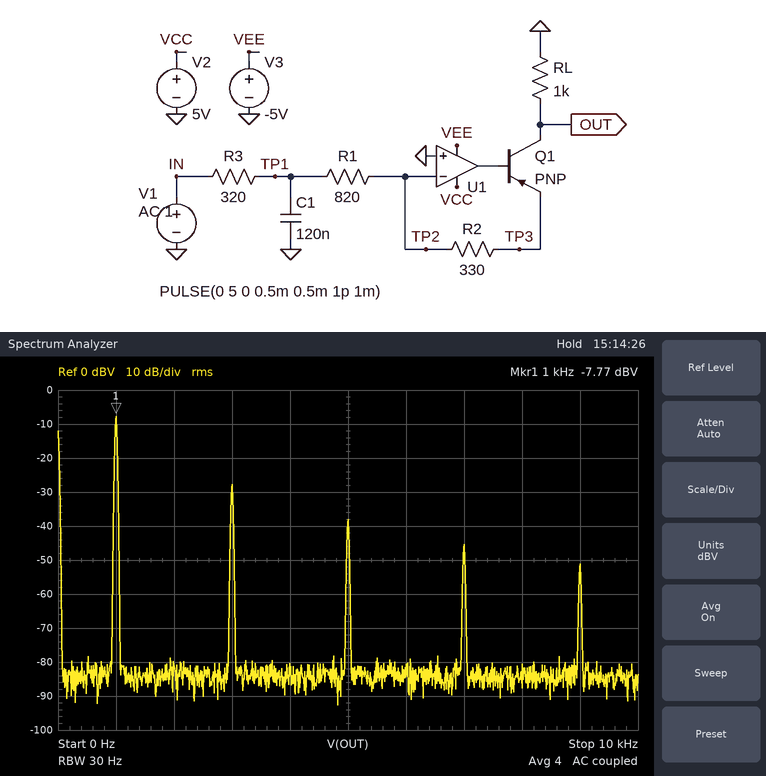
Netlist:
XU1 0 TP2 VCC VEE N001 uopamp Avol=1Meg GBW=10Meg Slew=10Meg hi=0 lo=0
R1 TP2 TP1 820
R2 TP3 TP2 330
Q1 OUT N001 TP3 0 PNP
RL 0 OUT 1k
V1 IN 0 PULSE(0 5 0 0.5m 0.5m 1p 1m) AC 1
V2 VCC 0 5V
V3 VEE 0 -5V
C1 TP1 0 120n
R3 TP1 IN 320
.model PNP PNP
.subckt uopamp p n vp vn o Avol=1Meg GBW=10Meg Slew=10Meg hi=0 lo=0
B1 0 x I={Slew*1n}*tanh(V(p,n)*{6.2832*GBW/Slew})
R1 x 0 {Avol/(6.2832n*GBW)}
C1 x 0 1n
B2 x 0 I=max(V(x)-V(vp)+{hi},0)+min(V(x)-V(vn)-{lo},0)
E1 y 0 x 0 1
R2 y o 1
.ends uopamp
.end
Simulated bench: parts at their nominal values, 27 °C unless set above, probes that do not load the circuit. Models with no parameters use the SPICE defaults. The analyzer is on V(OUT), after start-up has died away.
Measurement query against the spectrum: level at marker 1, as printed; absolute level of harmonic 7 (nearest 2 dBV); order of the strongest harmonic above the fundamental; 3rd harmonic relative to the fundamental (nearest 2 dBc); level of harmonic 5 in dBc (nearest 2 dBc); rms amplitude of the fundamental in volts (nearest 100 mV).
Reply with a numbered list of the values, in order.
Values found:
1. -7.77 dBV
2. -46 dBV
3. 3
4. -20 dBc
5. -30 dBc
6. 400 mV
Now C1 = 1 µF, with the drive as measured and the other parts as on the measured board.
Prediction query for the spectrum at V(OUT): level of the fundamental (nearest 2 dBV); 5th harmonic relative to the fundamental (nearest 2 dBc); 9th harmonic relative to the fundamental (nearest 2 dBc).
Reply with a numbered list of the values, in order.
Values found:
1. -12 dBV
2. -40 dBc
3. -56 dBc
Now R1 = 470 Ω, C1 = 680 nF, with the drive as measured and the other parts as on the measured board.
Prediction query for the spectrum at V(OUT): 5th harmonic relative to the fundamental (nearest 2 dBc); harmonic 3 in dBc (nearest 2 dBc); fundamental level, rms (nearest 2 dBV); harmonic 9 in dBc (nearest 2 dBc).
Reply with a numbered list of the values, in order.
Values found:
1. -38 dBc
2. -26 dBc
3. -6 dBV
4. -54 dBc
